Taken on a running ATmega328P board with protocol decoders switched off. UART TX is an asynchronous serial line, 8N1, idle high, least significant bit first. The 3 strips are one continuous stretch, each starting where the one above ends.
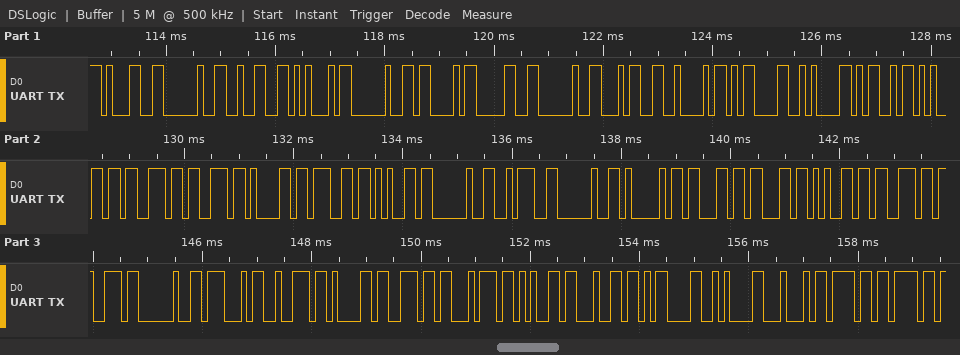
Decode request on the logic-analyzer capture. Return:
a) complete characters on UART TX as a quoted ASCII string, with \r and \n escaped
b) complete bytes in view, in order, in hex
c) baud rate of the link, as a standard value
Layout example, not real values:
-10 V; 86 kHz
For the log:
"1 2E C0 4B\r\nMessage : Access Granted\r\nDoo"; 31 20 32 45 20 43 30 20 34 42 0D 0A 4D 65 73 73 61 67 65 20 3A 20 41 63 63 65 73 73 20 47 72 61 6E 74 65 64 0D 0A 44 6F 6F; 9600 baud
